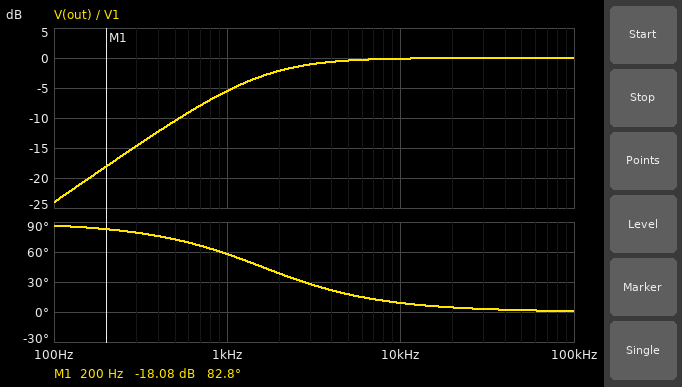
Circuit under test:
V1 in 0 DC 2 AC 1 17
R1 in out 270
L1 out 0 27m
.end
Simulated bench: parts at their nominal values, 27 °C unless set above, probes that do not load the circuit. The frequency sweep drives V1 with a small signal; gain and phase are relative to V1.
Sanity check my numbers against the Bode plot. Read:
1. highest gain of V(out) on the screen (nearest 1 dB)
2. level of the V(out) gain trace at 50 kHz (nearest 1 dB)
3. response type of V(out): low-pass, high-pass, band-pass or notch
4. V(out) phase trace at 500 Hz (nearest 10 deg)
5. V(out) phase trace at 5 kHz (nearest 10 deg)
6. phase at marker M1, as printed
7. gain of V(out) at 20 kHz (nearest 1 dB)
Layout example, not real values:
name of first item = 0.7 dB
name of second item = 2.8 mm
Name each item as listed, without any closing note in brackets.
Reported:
highest gain of V(out) on the screen = 0 dB
level of the V(out) gain trace at 50 kHz = 0 dB
response type of V(out): low-pass, high-pass, band-pass or notch = high-pass
V(out) phase trace at 500 Hz = 70 deg
V(out) phase trace at 5 kHz = 20 deg
phase at marker M1, as printed = 82.8 deg
gain of V(out) at 20 kHz = 0 dB
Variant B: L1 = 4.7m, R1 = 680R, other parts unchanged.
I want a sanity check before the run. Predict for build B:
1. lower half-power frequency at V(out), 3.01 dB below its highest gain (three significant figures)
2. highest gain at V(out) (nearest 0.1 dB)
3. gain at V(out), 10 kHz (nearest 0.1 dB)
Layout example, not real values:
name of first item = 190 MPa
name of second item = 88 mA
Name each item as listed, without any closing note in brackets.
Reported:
lower half-power frequency at V(out), 3.01 dB below its highest gain = 23.0 kHz
highest gain at V(out) = 0 dB
gain at V(out), 10 kHz = -8.0 dB
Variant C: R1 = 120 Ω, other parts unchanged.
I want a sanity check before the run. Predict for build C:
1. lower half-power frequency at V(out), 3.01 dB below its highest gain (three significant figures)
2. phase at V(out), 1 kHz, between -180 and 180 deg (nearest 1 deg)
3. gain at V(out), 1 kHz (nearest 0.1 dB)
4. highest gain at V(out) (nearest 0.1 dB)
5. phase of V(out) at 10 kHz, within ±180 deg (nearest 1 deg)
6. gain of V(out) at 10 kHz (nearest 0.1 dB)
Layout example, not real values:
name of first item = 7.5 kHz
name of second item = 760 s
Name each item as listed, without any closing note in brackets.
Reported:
lower half-power frequency at V(out), 3.01 dB below its highest gain = 707 Hz
phase at V(out), 1 kHz, between -180 and 180 deg = 35 deg
gain at V(out), 1 kHz = -1.8 dB
highest gain at V(out) = 0 dB
phase of V(out) at 10 kHz, within ±180 deg = 4 deg
gain of V(out) at 10 kHz = 0 dB
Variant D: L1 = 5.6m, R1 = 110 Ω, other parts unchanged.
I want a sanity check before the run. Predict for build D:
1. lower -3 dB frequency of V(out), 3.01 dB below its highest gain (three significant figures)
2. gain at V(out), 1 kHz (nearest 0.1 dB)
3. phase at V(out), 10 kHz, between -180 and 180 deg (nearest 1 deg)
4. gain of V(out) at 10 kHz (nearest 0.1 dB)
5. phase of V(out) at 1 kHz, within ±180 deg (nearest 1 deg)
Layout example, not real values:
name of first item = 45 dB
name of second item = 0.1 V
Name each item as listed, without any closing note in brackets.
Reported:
lower -3 dB frequency of V(out), 3.01 dB below its highest gain = 3.13 kHz
gain at V(out), 1 kHz = -10.3 dB
phase at V(out), 10 kHz, between -180 and 180 deg = 17 deg
gain of V(out) at 10 kHz = -0.4 dB
phase of V(out) at 1 kHz, within ±180 deg = 72 deg
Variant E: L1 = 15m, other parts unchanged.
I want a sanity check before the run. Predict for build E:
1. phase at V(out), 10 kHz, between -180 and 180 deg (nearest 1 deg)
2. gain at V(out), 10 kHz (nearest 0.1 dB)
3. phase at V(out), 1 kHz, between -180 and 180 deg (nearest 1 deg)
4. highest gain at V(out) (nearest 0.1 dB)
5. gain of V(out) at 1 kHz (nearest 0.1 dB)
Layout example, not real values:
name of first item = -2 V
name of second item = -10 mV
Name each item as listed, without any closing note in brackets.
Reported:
phase at V(out), 10 kHz, between -180 and 180 deg = 16 deg
gain at V(out), 10 kHz = -0.3 dB
phase at V(out), 1 kHz, between -180 and 180 deg = 71 deg
highest gain at V(out) = 0 dB
gain of V(out) at 1 kHz = -9.6 dB
